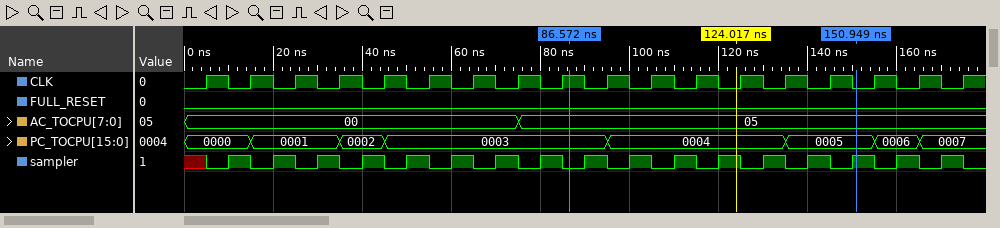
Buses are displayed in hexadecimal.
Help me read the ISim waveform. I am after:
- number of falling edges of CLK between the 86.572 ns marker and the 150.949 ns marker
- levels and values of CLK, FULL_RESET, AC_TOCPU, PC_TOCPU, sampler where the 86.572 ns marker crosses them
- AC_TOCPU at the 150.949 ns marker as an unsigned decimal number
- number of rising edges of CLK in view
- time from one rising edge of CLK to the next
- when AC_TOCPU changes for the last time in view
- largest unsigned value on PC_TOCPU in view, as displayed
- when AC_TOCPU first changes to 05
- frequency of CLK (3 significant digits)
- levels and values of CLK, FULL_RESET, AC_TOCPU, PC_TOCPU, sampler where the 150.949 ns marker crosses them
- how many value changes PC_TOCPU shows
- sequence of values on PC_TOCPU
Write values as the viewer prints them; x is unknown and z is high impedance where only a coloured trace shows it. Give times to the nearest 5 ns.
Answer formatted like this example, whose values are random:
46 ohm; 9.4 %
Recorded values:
7; CLK=1, FULL_RESET=0, AC_TOCPU=05, PC_TOCPU=0003, sampler=0; 5; 18; 10 ns; 75 ns; 0007; 75 ns; 100 MHz; CLK=0, FULL_RESET=0, AC_TOCPU=05, PC_TOCPU=0005, sampler=1; 7; 0000, 0001, 0002, 0003, 0004, 0005, 0006, 0007
